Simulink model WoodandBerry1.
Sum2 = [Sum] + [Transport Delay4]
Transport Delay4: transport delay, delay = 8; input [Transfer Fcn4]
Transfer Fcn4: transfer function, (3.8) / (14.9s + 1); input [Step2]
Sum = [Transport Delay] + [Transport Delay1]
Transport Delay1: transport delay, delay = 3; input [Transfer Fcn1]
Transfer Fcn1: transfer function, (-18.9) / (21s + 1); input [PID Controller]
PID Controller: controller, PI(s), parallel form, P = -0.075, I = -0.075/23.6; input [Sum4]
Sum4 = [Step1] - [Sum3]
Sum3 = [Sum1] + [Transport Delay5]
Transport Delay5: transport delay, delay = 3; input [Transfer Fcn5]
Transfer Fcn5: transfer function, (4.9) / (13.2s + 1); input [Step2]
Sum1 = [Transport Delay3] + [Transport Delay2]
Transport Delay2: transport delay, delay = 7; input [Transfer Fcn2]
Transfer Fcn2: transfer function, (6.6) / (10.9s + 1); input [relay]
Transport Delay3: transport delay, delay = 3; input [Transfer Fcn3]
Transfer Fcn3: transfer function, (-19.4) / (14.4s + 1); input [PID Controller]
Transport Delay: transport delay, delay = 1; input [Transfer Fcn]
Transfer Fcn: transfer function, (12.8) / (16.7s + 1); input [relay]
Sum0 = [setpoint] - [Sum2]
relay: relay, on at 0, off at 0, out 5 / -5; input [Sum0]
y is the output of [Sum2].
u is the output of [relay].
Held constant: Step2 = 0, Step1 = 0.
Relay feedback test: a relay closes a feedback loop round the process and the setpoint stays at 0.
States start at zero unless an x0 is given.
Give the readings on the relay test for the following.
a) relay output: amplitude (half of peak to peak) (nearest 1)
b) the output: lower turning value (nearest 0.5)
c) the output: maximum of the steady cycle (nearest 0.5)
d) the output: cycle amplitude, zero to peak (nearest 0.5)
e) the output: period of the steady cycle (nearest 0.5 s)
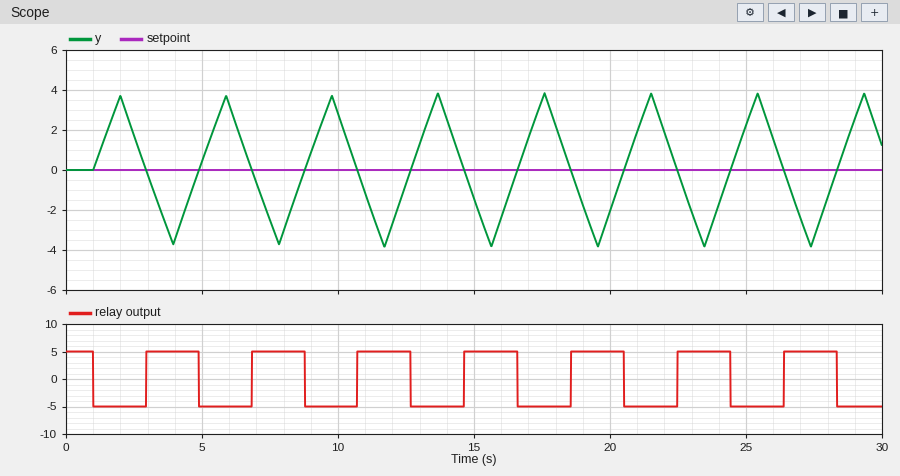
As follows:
5
-4.0
4.0
4.0
4.0 s
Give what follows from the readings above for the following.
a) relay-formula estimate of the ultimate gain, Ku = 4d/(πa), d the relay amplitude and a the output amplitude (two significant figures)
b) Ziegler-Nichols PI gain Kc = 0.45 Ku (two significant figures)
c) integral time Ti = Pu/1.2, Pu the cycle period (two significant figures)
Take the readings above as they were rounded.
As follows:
1.6
0.72
3.3 s
